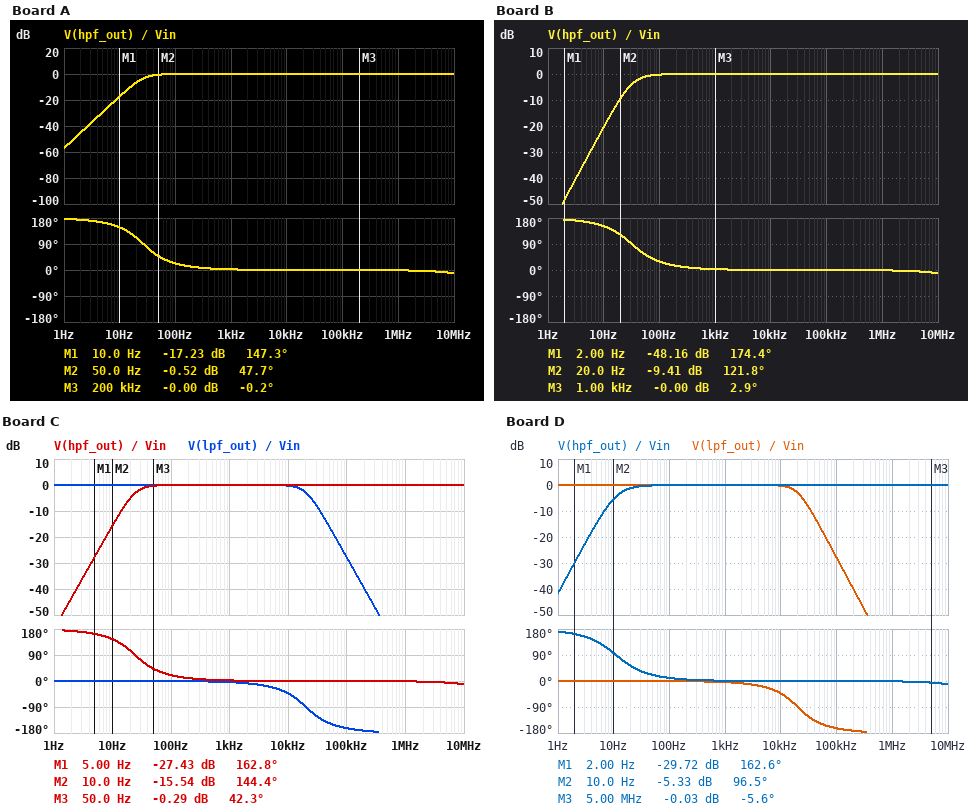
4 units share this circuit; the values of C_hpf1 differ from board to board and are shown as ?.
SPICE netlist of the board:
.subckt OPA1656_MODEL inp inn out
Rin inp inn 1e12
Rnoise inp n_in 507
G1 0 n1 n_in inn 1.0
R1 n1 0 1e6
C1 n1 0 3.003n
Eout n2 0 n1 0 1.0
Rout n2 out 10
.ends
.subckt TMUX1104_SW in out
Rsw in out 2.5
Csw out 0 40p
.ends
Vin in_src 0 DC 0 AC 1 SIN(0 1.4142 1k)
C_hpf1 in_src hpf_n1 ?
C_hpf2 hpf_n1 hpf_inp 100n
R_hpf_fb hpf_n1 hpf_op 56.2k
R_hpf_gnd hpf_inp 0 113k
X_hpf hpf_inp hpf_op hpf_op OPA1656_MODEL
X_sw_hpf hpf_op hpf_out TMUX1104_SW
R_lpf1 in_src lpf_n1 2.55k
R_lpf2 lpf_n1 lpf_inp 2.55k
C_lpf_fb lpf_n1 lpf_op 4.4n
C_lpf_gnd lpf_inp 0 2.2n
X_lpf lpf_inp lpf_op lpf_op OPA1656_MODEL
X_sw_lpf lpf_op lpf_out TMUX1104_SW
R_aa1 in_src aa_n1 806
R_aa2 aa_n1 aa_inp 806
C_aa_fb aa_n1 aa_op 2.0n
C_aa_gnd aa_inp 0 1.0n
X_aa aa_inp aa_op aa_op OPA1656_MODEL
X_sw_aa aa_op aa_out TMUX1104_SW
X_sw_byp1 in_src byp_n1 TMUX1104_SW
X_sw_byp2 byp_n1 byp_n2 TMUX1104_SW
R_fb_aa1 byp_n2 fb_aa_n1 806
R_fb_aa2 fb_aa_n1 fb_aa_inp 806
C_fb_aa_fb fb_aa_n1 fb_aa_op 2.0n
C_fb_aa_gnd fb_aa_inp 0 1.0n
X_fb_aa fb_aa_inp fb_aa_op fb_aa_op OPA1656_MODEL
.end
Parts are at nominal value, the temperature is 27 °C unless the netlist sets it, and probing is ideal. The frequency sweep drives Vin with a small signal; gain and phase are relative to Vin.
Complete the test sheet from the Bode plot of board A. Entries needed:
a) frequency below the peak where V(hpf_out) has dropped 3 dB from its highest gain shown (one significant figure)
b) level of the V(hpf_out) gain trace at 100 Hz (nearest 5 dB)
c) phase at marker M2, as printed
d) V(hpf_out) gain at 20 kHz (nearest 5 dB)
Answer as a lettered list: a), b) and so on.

a) 30 Hz
b) 0 dB
c) 47.7 deg
d) 0 dB
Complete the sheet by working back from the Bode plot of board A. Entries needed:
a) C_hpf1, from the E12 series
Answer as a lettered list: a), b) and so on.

a) 56 nF
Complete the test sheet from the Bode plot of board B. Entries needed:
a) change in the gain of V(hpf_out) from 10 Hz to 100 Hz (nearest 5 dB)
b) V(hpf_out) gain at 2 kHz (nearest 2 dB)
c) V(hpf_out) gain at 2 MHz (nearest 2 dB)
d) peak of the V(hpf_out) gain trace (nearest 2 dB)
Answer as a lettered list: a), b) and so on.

a) 20 dB
b) 0 dB
c) 0 dB
d) 0 dB
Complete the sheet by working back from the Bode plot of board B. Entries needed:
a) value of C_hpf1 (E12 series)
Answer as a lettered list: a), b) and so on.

a) 39 nF
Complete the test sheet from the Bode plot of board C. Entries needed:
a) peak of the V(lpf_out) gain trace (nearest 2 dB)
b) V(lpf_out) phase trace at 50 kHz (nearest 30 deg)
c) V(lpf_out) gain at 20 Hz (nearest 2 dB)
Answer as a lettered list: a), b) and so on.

a) 0 dB
b) -150 deg
c) 0 dB
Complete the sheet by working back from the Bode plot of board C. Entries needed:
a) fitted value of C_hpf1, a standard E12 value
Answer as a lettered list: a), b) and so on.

a) 68 nF
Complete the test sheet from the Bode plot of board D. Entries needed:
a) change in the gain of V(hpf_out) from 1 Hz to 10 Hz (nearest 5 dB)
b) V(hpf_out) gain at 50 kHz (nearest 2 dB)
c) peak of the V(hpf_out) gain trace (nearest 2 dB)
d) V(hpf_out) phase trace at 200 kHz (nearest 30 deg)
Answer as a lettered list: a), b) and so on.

a) 35 dB
b) 0 dB
c) 0 dB
d) 0 deg
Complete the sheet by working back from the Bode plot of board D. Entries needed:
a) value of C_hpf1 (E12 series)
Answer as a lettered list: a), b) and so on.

a) 330 nF
